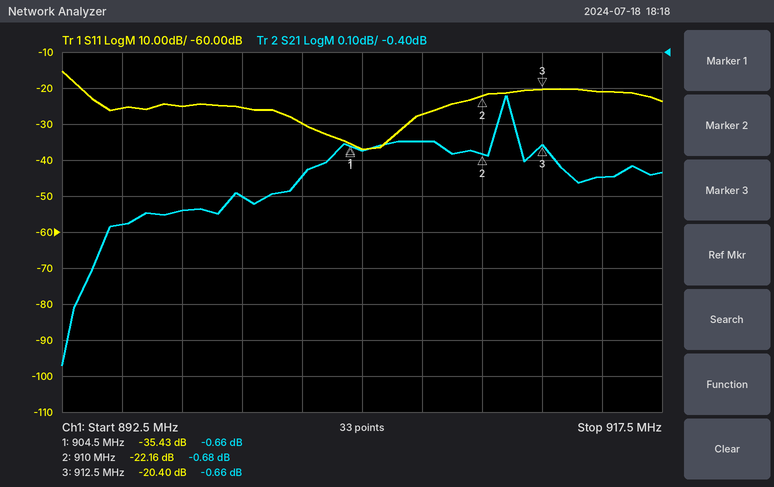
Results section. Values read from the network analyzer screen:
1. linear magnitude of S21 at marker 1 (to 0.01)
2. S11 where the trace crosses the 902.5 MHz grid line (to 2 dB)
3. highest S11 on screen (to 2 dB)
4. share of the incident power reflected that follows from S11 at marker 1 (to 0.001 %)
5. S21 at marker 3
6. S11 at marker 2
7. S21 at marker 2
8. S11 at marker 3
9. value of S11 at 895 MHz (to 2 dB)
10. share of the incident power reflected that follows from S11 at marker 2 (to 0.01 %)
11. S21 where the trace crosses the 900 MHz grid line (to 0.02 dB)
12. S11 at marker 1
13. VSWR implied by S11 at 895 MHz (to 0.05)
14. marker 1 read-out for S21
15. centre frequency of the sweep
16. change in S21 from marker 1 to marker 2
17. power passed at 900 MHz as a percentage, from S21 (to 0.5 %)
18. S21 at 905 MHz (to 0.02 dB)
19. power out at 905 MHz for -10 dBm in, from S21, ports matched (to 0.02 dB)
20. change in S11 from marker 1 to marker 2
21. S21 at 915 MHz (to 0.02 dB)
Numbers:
0.93
-30 dB
-16 dB
0.029 %
-0.66 dB
-22.16 dB
-0.68 dB
-20.40 dB
-26 dB
0.61 %
-0.80 dB
-35.43 dB
1.10
-0.66 dB
905 MHz
-0.02 dB
83.0 %
-0.68 dB
-10.68 dBm
13.27 dB
-0.74 dB
